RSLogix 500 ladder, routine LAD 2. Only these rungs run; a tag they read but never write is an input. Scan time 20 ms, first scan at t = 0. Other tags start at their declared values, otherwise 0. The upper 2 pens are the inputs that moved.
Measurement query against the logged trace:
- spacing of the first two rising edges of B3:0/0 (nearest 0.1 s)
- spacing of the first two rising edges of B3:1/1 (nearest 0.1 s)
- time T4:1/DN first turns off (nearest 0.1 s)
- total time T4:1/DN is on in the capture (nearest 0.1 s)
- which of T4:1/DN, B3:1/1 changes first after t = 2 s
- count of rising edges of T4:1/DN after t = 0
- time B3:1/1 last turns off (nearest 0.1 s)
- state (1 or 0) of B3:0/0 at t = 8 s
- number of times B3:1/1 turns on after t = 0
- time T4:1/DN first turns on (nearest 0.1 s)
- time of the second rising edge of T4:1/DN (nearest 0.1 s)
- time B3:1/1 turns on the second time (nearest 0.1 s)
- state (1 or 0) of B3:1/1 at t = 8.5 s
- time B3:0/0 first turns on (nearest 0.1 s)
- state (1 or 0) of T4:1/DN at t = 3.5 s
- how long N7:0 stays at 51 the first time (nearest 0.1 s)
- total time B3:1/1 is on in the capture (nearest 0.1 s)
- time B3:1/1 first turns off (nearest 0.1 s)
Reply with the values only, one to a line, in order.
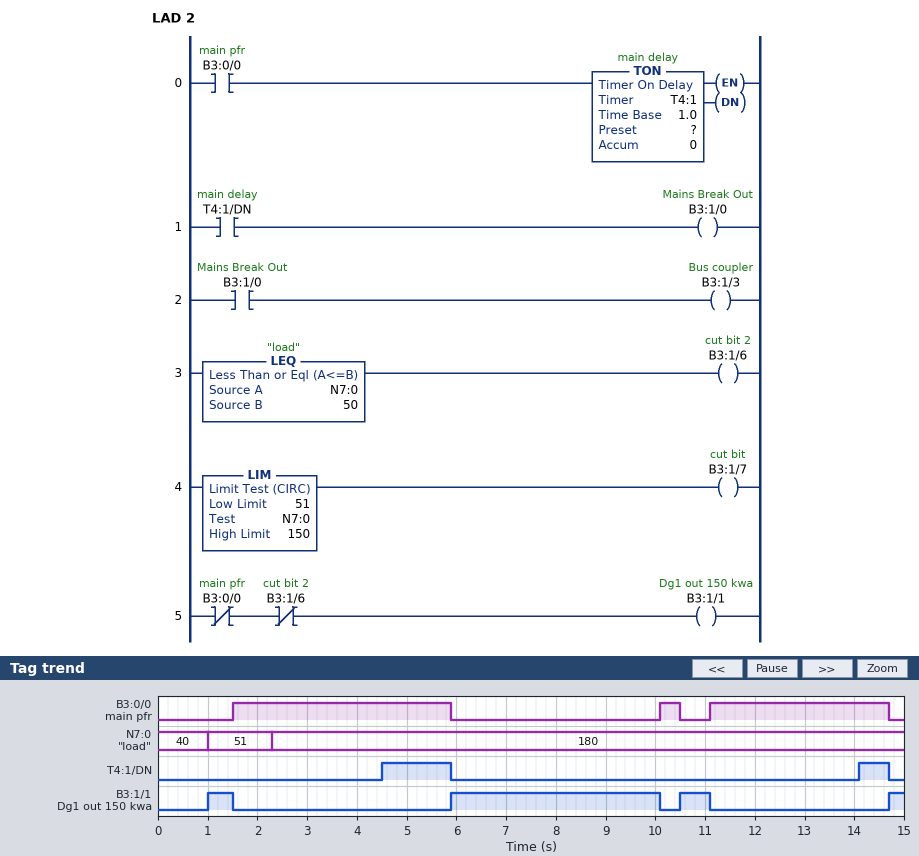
8.6 s
4.9 s
5.9 s
2.0 s
T4:1/DN
2
11.1 s
0
4
4.5 s
14.1 s
5.9 s
1
1.5 s
0
1.3 s
5.6 s
1.5 s
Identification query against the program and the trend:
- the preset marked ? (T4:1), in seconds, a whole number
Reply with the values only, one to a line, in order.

3 s
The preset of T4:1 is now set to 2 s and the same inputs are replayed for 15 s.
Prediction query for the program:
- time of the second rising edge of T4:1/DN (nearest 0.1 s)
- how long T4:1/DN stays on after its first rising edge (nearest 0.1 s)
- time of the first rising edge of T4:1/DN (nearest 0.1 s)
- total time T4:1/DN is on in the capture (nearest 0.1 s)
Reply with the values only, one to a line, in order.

13.1 s
2.4 s
3.5 s
4.0 s
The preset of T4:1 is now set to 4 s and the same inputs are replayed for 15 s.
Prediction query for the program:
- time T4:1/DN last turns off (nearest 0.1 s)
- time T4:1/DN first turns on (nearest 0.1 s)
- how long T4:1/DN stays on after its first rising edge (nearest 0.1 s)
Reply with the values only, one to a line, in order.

5.9 s
5.5 s
0.4 s
